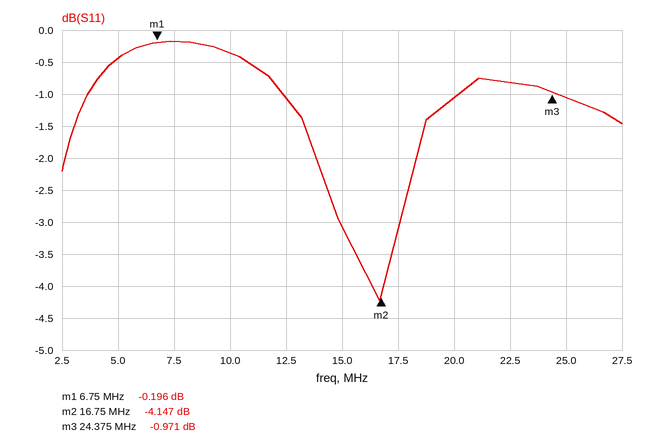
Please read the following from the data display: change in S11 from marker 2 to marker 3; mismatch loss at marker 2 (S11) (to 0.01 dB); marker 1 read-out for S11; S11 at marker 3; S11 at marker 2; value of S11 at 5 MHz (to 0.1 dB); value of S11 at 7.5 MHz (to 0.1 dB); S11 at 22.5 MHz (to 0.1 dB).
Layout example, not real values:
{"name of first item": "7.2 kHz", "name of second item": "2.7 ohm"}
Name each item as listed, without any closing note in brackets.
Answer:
{"change in S11 from marker 2 to marker 3": "3.176 dB", "mismatch loss at marker 2 (S11)": "2.11 dB", "marker 1 read-out for S11": "-0.196 dB", "S11 at marker 3": "-0.971 dB", "S11 at marker 2": "-4.147 dB", "value of S11 at 5 MHz": "-0.4 dB", "value of S11 at 7.5 MHz": "-0.2 dB", "S11 at 22.5 MHz": "-0.8 dB"}
